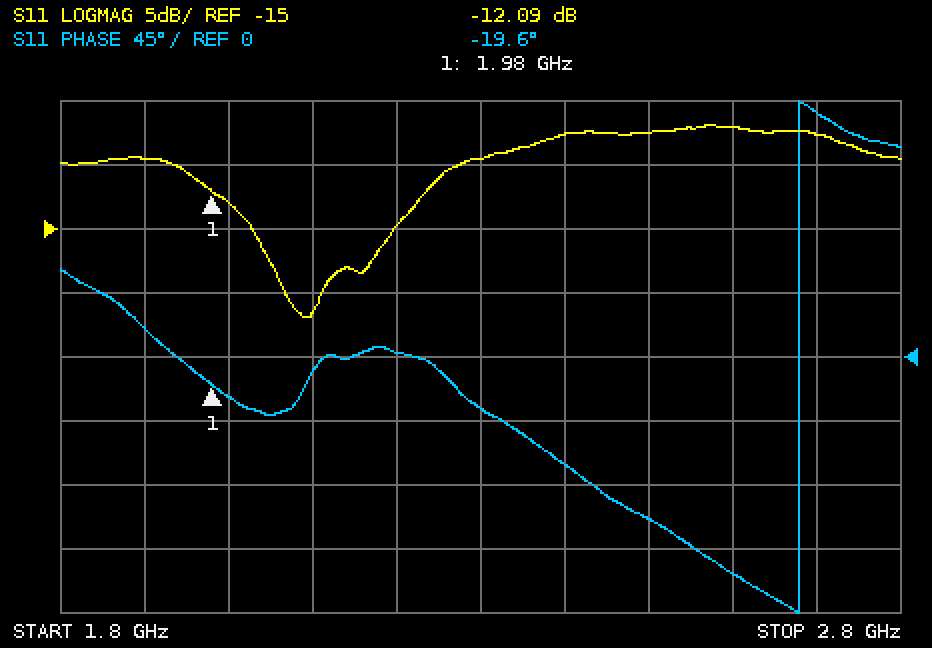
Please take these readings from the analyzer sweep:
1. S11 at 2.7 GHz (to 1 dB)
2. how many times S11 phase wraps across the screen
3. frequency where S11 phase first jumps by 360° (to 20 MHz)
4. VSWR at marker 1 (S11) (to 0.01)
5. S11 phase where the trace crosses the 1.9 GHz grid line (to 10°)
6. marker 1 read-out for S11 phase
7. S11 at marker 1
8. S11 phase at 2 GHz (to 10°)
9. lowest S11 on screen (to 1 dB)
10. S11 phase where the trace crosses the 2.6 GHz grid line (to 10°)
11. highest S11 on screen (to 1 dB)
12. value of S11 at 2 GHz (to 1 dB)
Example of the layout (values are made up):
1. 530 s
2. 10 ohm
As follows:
1. -8 dB
2. 1
3. 2.68 GHz
4. 1.66
5. 20°
6. -19.6°
7. -12.09 dB
8. -30°
9. -22 dB
10. -150°
11. -7 dB
12. -13 dB
